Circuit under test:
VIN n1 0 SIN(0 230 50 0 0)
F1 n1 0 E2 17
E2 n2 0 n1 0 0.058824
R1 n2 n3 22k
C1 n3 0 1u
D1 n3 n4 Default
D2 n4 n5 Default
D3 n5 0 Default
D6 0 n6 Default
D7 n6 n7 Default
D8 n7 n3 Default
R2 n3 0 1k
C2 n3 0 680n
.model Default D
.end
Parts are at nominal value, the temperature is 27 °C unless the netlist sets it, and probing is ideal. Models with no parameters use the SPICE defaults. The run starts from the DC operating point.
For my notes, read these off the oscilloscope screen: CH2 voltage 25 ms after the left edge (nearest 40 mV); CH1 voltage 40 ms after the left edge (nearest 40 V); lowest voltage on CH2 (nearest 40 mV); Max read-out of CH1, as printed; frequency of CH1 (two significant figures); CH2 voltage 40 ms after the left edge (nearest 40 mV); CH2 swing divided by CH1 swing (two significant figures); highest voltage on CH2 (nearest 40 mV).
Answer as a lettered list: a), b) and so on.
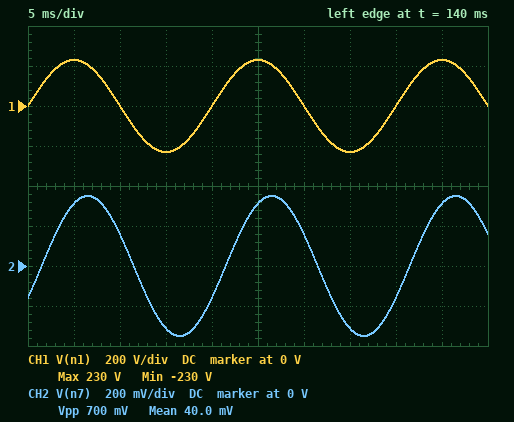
a) 320 mV
b) 0 V
c) -360 mV
d) 230 V
e) 50 Hz
f) -160 mV
g) 0.0015
h) 360 mV
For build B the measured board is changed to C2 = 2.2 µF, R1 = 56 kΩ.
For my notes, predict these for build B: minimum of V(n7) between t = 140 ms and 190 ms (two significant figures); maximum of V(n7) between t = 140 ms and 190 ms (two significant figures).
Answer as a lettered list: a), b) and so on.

a) -110 mV
b) 110 mV
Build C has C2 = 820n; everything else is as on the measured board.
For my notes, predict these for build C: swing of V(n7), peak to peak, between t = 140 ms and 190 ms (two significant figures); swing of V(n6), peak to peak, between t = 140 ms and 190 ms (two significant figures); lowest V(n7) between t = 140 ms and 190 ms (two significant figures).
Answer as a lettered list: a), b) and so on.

a) 690 mV
b) 340 mV
c) -340 mV
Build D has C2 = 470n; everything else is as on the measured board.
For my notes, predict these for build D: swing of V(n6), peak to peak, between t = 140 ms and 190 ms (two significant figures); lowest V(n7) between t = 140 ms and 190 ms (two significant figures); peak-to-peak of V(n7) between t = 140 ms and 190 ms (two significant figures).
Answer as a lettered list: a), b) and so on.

a) 360 mV
b) -360 mV
c) 720 mV
